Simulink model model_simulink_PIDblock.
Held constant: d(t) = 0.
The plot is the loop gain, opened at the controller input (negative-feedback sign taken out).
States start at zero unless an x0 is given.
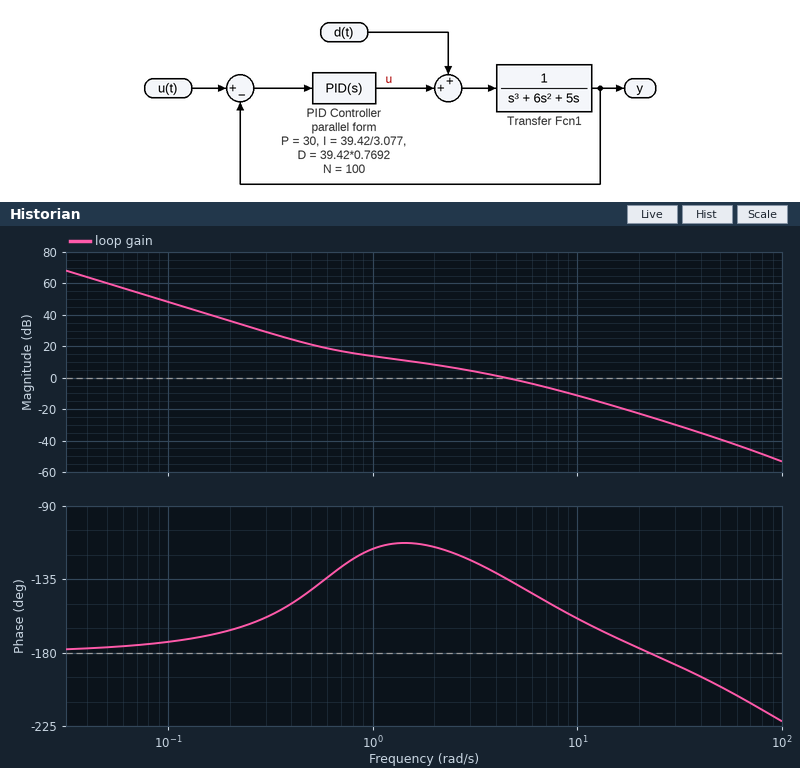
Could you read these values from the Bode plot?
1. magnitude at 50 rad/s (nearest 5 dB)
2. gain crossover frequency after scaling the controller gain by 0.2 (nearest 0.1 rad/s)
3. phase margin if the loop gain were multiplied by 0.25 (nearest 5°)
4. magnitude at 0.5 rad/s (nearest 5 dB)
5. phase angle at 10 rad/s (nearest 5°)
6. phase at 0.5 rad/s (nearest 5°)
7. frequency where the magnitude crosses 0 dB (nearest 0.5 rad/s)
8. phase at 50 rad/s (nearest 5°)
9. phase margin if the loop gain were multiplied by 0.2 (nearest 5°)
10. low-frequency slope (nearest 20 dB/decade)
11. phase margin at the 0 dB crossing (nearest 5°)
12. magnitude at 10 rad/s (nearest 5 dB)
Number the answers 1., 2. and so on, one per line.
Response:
1. -40 dB
2. 1.0 rad/s
3. 65°
4. 20 dB
5. -160°
6. -140°
7. 4.5 rad/s
8. -200°
9. 65°
10. -40 dB/decade
11. 45°
12. -10 dB
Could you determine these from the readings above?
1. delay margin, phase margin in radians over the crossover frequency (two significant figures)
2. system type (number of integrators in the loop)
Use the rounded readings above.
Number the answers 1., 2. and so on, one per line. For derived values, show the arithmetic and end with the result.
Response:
1. 45 × π / 180 / 4.5 = 0.17 s
2. 2
